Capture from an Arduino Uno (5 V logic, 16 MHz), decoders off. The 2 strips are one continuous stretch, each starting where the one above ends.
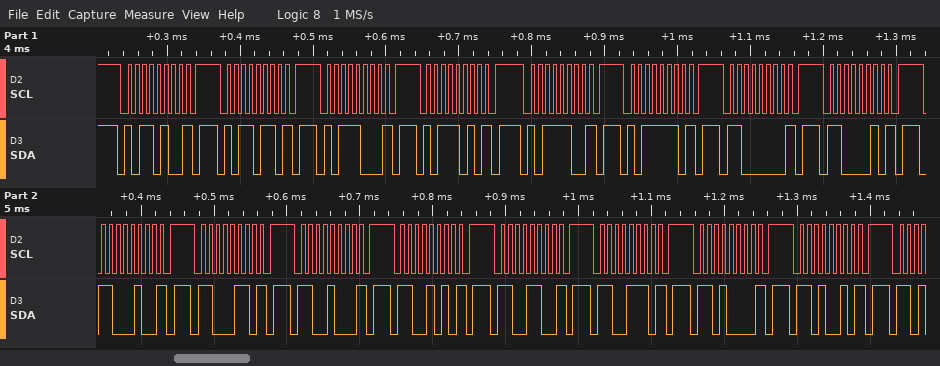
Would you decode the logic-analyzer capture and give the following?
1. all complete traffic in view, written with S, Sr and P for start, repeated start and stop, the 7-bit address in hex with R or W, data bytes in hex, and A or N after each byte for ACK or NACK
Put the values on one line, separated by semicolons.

S 5AW N P S 5BW N P S 5CW N P S 5DW N P S 5EW N P S 5FW N P S 60W N P S 61W N P S 62W N P S 63W N P S 64W N P S 65W N P S 66W N P S 67W N P S 68W N P S 69W N P
